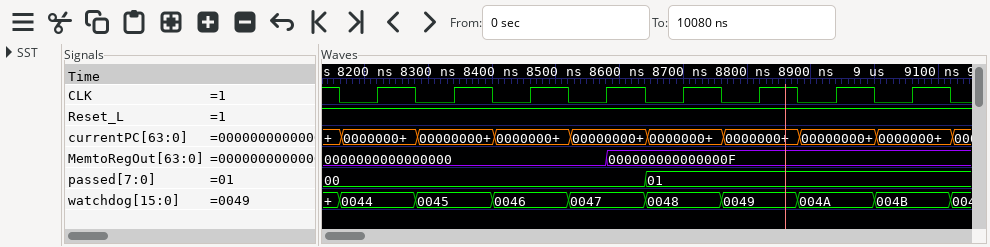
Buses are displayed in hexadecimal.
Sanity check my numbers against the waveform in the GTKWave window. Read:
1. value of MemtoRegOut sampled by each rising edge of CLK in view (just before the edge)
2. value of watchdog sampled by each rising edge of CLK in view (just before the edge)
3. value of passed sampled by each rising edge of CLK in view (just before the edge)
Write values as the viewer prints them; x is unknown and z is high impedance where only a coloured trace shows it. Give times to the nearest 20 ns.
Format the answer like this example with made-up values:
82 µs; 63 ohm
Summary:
0000000000000000, 0000000000000000, 0000000000000000, 0000000000000000, 000000000000000F, 000000000000000F, 000000000000000F, 000000000000000F; 0044, 0045, 0046, 0047, 0048, 0049, 004A, 004B; 00, 00, 00, 00, 01, 01, 01, 01
